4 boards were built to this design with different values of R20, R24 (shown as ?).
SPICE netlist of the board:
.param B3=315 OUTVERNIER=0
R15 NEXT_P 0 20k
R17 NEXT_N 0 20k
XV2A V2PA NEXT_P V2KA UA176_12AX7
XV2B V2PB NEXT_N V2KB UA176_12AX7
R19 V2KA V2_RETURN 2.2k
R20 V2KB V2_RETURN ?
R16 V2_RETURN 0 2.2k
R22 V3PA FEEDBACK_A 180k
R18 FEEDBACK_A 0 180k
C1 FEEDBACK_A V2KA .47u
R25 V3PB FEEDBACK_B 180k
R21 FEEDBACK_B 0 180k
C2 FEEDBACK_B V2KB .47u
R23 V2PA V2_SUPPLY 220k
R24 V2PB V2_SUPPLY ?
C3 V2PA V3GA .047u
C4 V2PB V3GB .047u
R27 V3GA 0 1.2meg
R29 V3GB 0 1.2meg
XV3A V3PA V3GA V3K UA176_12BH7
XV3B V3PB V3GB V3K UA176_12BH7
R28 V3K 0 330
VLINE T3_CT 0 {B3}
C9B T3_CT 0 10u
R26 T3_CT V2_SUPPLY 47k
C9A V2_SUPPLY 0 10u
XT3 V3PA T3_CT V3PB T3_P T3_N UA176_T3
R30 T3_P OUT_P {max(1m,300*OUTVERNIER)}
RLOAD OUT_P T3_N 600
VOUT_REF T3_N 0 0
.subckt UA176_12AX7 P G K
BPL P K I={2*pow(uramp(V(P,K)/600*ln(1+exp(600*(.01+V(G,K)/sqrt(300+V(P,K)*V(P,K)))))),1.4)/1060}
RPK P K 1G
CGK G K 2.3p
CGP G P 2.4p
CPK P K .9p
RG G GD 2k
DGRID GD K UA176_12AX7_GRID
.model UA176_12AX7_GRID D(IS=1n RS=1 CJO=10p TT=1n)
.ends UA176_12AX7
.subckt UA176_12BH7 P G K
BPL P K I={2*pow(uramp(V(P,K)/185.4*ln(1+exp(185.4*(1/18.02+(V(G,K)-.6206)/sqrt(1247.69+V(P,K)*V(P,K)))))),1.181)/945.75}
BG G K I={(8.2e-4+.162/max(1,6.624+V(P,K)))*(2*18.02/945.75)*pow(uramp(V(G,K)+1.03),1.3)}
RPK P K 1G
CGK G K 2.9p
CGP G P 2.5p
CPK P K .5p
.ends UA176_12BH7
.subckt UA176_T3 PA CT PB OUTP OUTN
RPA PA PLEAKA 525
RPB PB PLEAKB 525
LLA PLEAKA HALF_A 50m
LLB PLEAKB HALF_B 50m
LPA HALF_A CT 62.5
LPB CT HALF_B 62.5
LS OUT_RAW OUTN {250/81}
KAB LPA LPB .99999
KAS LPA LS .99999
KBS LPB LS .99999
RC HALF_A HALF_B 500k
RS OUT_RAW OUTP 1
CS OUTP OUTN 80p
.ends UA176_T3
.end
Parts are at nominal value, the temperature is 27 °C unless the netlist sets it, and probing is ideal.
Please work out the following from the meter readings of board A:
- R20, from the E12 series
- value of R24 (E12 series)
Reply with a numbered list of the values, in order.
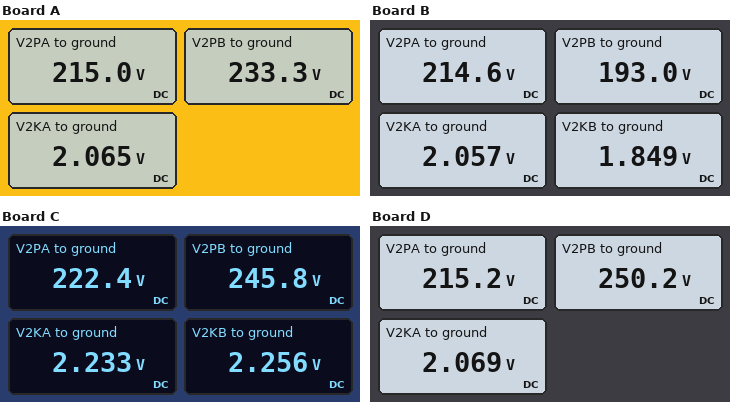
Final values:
1. 3.3 kΩ
2. 180 kΩ
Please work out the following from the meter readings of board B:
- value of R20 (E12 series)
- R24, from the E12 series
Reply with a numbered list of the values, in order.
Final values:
1. 1.8 kΩ
2. 330 kΩ
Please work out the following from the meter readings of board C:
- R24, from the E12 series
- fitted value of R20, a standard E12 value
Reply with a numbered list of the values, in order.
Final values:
1. 68 kΩ
2. 1.2 kΩ
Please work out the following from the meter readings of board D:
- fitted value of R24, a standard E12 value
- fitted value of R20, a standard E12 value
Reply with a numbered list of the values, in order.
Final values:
1. 120 kΩ
2. 3.9 kΩ
